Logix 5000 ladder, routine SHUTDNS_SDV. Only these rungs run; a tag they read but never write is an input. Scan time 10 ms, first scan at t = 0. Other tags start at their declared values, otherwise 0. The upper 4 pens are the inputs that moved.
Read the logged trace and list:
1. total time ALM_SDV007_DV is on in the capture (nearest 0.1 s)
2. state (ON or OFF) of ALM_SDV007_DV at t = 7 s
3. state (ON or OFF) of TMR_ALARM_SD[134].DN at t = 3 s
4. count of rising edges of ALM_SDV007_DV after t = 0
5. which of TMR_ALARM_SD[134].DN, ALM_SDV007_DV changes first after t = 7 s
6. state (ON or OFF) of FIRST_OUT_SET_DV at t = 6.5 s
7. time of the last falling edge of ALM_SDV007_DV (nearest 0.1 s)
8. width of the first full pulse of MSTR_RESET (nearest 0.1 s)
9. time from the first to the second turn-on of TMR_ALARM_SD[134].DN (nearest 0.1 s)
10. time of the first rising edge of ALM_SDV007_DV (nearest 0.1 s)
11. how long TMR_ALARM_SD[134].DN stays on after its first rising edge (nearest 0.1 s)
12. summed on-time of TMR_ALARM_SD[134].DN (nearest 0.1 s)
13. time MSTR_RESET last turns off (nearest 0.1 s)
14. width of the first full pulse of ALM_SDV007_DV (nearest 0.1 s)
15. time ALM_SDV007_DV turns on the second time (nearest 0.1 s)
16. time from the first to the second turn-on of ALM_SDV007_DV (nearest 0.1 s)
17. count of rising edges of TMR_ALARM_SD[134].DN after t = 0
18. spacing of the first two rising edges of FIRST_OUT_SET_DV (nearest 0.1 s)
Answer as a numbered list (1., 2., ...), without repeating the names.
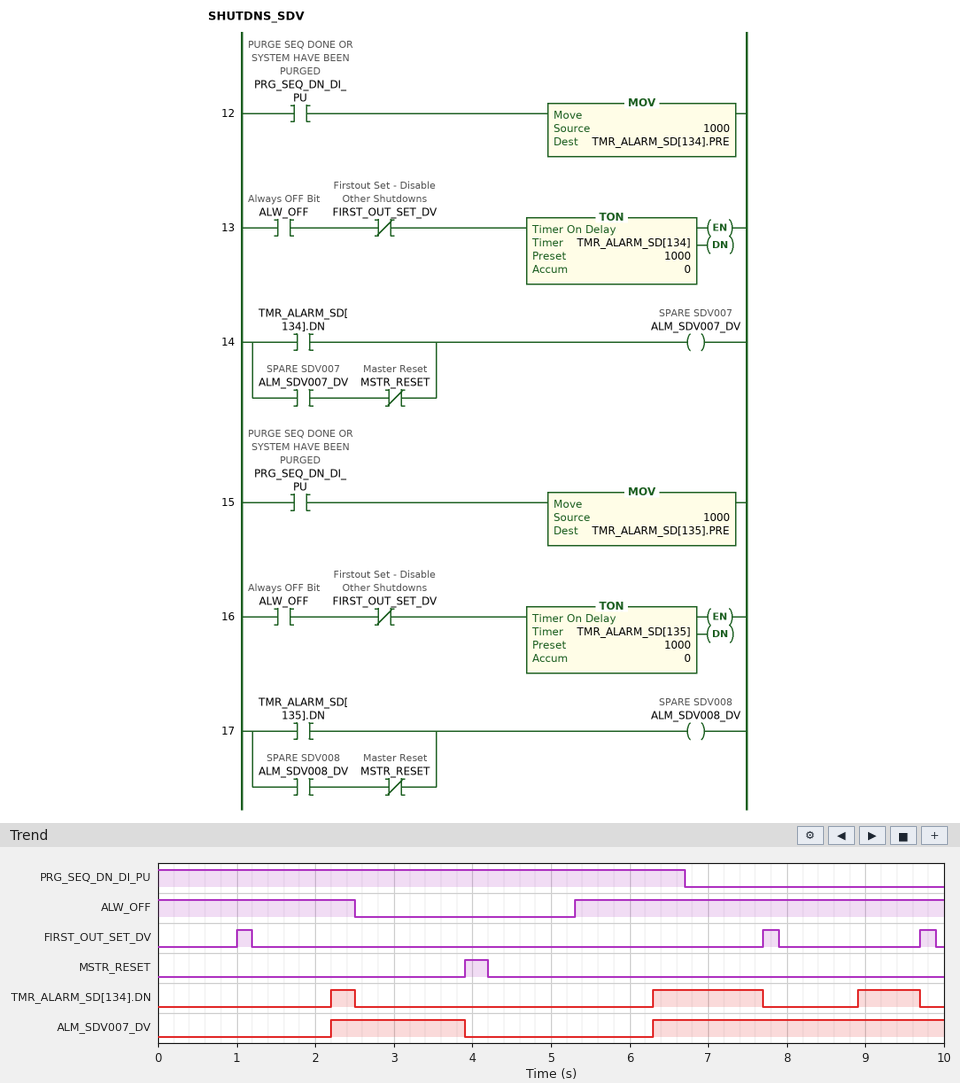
1. 5.4 s
2. ON
3. OFF
4. 2
5. TMR_ALARM_SD[134].DN
6. OFF
7. 3.9 s
8. 0.3 s
9. 4.1 s
10. 2.2 s
11. 0.3 s
12. 2.5 s
13. 4.2 s
14. 1.7 s
15. 6.3 s
16. 4.1 s
17. 3
18. 6.7 s
